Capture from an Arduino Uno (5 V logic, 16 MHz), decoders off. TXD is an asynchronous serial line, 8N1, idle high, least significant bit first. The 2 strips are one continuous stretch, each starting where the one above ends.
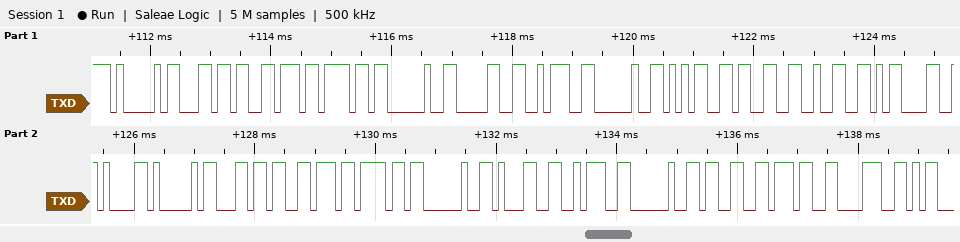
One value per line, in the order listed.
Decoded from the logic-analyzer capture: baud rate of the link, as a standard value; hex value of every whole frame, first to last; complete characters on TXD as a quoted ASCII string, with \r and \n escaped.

9600 baud
41 6C 76 6F 20 30 3A 20 35 33 32 0D 0A 41 6C 76 6F 20 31 3A 20 33 37 38
"Alvo 0: 532\r\nAlvo 1: 378"
